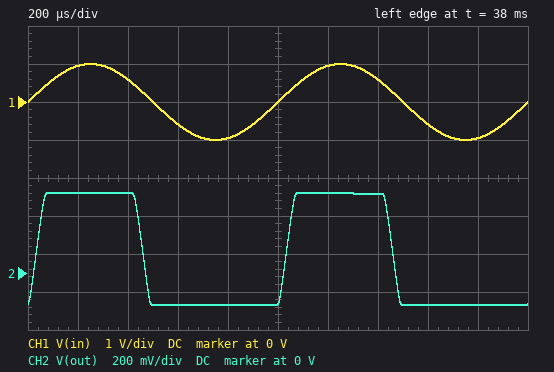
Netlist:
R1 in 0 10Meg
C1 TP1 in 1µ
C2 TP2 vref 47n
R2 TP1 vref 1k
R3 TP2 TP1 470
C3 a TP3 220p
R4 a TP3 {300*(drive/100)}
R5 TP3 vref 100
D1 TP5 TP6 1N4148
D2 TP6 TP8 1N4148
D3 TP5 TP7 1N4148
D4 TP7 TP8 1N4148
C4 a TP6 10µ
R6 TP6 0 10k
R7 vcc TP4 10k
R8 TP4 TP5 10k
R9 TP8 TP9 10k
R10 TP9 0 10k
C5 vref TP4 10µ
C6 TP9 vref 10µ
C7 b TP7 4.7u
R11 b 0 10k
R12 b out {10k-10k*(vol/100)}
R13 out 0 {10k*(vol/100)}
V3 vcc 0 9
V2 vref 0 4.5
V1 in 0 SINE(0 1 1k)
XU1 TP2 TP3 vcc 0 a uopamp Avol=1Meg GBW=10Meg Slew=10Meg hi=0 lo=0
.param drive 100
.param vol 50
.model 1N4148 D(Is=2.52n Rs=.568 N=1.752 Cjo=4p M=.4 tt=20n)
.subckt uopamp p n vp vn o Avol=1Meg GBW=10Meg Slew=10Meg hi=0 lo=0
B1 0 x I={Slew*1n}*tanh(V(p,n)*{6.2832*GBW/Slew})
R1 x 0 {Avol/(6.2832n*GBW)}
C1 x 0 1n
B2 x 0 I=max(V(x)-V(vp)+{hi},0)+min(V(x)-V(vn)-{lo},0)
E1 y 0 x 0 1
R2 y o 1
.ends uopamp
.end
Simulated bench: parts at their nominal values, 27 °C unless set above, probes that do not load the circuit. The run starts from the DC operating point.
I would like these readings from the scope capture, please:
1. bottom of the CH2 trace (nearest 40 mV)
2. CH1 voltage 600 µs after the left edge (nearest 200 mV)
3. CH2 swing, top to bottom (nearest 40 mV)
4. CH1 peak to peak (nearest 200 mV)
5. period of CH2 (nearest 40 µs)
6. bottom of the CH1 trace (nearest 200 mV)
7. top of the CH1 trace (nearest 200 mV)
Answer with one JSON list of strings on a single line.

["-160 mV", "-600 mV", "600 mV", "2.0 V", "1.00 ms", "-1.0 V", "1.0 V"]
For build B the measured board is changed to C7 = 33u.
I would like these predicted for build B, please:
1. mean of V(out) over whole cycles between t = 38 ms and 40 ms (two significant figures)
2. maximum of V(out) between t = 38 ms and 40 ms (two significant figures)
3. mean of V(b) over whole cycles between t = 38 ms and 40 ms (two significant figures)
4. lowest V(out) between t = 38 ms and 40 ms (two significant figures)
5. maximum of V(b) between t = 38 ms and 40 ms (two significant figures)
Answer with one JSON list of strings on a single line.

["140 mV", "470 mV", "270 mV", "-120 mV", "940 mV"]
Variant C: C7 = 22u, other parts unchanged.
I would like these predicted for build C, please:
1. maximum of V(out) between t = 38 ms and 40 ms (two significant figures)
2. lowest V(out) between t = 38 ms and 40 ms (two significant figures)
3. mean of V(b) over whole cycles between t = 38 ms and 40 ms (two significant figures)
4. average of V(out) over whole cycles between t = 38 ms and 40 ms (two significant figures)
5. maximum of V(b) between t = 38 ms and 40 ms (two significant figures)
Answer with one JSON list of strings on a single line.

["460 mV", "-130 mV", "260 mV", "130 mV", "930 mV"]
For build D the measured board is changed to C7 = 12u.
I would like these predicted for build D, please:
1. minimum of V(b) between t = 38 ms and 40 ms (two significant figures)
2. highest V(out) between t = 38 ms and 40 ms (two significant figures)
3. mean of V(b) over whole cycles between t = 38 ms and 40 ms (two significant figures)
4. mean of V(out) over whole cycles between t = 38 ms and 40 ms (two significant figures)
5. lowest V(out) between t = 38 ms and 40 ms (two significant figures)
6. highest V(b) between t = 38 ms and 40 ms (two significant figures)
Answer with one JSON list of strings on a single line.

["-280 mV", "450 mV", "230 mV", "120 mV", "-140 mV", "900 mV"]
